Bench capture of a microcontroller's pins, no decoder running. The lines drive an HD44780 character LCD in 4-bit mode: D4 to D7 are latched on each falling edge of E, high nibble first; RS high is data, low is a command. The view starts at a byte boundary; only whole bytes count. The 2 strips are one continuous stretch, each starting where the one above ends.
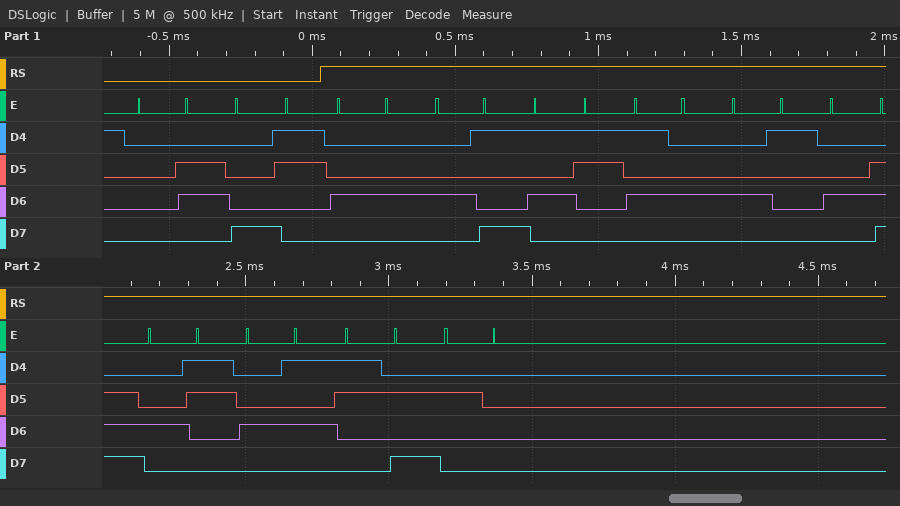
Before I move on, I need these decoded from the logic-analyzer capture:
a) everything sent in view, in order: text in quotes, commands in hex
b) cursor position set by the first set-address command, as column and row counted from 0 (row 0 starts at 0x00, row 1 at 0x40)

0x06 0x83 "DISTANCE: "
column 3, row 0
